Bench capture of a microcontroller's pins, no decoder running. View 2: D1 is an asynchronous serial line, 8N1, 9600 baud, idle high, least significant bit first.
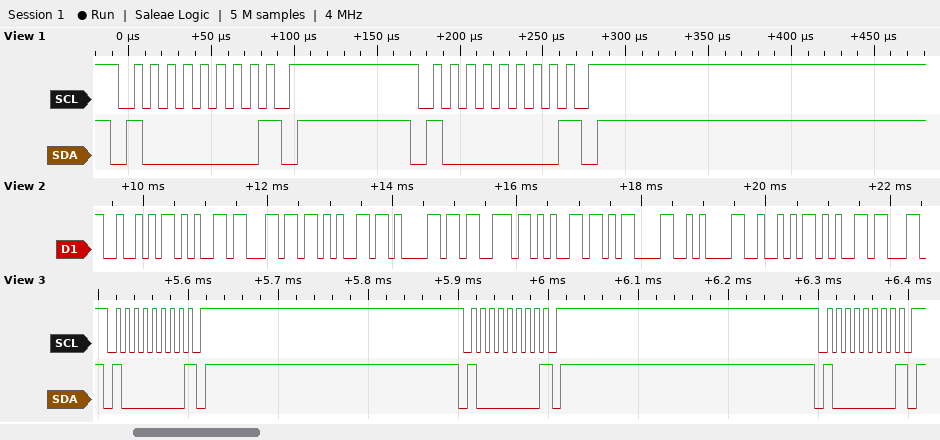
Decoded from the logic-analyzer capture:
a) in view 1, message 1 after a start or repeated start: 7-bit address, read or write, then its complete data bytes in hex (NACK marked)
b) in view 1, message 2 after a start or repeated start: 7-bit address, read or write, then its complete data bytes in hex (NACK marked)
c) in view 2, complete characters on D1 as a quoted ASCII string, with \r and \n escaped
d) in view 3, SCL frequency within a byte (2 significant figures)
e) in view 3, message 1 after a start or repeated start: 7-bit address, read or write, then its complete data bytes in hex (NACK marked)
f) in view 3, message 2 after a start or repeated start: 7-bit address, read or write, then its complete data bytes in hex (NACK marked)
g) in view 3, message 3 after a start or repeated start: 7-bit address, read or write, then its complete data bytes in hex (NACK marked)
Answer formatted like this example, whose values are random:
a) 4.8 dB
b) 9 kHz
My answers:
a) 0x40 write NACK
b) 0x40 write NACK
c) "Release\r\nRe"
d) 100 kHz
e) 0x40 write NACK
f) 0x40 write NACK
g) 0x40 write NACK
